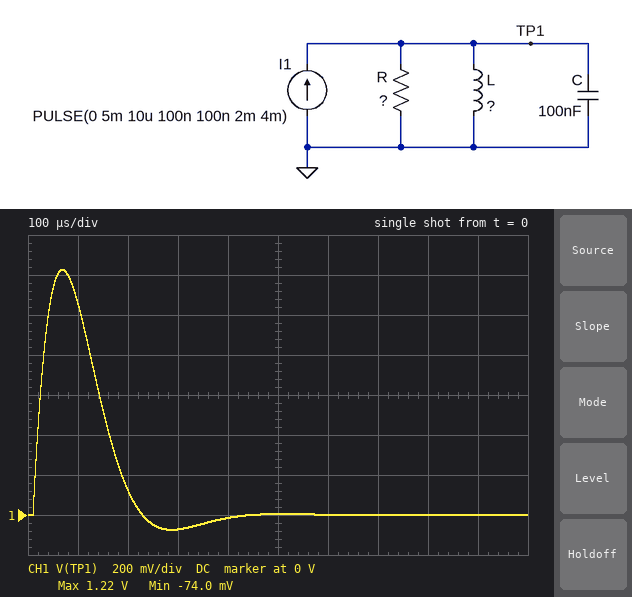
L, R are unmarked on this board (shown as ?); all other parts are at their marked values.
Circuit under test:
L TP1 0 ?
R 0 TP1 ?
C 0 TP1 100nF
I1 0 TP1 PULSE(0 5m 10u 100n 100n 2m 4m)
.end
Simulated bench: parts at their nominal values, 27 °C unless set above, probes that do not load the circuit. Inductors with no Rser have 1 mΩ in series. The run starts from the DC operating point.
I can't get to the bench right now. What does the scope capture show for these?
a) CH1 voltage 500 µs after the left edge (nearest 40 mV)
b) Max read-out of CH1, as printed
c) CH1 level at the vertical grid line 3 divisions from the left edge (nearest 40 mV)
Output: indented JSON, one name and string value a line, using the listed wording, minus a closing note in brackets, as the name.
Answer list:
{
  "CH1 voltage 500 µs after the left edge": "0 V",
  "Max read-out of CH1, as printed": "1.22 V",
  "CH1 level at the vertical grid line 3 divisions from the left edge": "-80 mV"
}
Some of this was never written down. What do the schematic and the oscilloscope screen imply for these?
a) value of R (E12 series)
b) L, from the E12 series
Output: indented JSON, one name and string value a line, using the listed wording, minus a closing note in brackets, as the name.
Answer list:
{
  "value of R": "390 Ω",
  "L, from the E12 series": "27 mH"
}
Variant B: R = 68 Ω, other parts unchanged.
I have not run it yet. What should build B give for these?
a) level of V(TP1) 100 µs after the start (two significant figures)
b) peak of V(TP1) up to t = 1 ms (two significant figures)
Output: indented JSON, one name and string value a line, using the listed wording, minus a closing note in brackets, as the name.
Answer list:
{
  "level of V(TP1) 100 µs after the start": "280 mV",
  "peak of V(TP1) up to t = 1 ms": "320 mV"
}
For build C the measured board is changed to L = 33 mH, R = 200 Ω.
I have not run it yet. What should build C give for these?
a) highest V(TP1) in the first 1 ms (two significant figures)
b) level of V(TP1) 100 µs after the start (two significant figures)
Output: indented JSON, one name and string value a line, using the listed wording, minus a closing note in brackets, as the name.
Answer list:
{
  "highest V(TP1) in the first 1 ms": "820 mV",
  "level of V(TP1) 100 µs after the start": "710 mV"
}
